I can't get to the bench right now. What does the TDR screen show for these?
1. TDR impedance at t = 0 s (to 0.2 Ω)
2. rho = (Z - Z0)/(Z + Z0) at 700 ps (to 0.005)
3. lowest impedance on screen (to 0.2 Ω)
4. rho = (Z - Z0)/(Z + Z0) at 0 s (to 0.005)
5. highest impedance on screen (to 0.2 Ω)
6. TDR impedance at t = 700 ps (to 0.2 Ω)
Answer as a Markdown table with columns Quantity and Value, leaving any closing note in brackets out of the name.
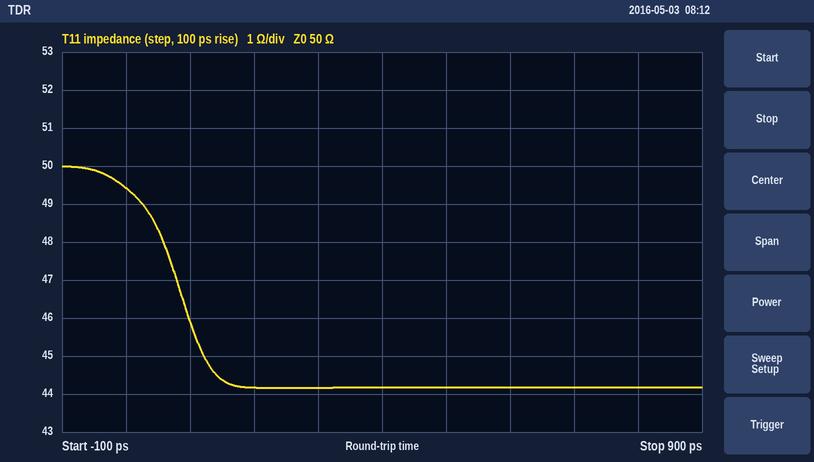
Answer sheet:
| Quantity | Value |
|---|---|
| TDR impedance at t = 0 s | 49.4 Ω |
| rho = (Z - Z0)/(Z + Z0) at 700 ps | -0.060 |
| lowest impedance on screen | 44.2 Ω |
| rho = (Z - Z0)/(Z + Z0) at 0 s | -0.005 |
| highest impedance on screen | 50.0 Ω |
| TDR impedance at t = 700 ps | 44.2 Ω |
